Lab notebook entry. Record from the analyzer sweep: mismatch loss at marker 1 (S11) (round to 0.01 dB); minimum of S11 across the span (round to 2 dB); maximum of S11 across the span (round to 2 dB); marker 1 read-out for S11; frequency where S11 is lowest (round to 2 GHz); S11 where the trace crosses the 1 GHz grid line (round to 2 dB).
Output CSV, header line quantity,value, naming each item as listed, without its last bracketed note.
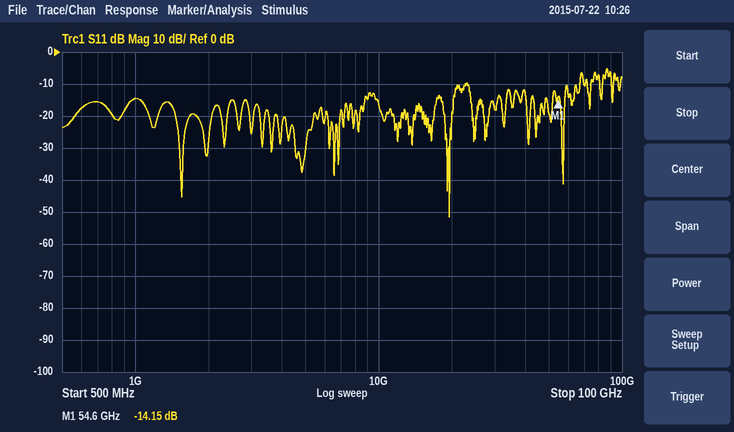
quantity,value
mismatch loss at marker 1 (S11),0.17 dB
minimum of S11 across the span,-52 dB
maximum of S11 across the span,-6 dB
marker 1 read-out for S11,-14.15 dB
frequency where S11 is lowest,20 GHz
S11 where the trace crosses the 1 GHz grid line,-14 dB
